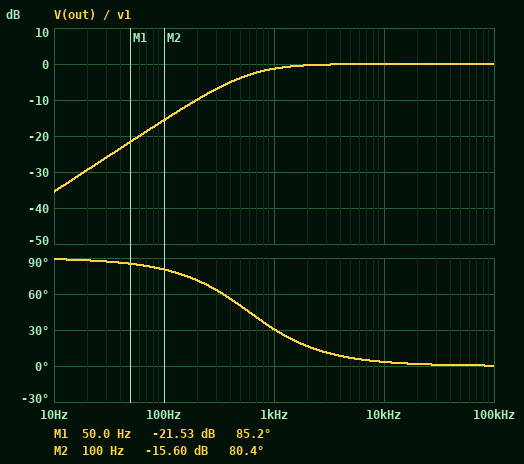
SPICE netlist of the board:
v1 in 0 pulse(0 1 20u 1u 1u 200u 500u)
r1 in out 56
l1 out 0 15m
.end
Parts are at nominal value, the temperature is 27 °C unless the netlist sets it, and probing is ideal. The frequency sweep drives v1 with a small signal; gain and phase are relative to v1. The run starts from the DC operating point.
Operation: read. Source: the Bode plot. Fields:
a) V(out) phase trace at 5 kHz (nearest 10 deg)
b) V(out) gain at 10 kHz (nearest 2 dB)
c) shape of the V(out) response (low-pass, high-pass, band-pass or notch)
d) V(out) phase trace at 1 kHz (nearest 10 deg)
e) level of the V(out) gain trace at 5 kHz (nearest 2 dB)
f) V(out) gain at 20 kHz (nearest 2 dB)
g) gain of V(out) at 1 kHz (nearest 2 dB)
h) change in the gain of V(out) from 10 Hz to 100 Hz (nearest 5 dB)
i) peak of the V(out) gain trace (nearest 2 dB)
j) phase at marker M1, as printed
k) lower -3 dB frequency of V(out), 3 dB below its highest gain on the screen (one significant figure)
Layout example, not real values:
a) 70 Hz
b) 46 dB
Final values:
a) 10 deg
b) 0 dB
c) high-pass
d) 30 deg
e) 0 dB
f) 0 dB
g) -2 dB
h) 20 dB
i) 0 dB
j) 85.2 deg
k) 600 Hz
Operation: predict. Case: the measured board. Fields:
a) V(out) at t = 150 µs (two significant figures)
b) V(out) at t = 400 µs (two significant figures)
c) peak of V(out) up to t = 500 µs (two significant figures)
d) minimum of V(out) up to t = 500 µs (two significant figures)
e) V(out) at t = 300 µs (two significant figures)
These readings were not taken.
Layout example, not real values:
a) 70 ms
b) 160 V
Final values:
a) 620 mV
b) -270 mV
c) 1.0 V
d) -530 mV
e) -390 mV
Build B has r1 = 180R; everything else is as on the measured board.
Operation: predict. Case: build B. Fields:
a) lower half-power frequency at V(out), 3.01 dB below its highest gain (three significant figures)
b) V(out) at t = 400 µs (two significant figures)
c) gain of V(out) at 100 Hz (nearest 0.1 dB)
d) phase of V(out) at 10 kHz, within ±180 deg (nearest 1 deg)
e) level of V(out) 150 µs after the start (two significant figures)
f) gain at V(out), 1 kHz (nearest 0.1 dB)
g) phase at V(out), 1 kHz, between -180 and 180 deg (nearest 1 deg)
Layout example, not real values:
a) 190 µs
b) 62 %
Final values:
a) 1.91 kHz
b) -110 mV
c) -25.6 dB
d) 11 deg
e) 210 mV
f) -6.7 dB
g) 62 deg
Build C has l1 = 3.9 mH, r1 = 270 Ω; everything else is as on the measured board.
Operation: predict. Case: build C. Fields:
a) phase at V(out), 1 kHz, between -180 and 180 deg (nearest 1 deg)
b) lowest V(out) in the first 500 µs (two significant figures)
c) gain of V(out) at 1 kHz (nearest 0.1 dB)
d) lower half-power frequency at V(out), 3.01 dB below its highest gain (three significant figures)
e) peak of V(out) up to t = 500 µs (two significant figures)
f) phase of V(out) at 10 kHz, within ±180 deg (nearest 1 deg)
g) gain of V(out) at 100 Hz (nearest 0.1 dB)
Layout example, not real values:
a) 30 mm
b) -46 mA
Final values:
a) 85 deg
b) -970 mV
c) -20.9 dB
d) 11.0 kHz
e) 970 mV
f) 48 deg
g) -40.8 dB
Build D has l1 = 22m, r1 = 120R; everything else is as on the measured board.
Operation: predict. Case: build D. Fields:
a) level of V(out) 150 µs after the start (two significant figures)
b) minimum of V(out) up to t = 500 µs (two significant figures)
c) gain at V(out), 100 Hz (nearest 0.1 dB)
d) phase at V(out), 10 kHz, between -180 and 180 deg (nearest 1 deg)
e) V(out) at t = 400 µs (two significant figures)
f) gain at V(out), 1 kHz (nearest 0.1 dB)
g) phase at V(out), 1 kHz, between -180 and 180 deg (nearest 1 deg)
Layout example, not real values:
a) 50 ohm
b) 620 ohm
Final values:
a) 490 mV
b) -660 mV
c) -18.8 dB
d) 5 deg
e) -250 mV
f) -2.4 dB
g) 41 deg
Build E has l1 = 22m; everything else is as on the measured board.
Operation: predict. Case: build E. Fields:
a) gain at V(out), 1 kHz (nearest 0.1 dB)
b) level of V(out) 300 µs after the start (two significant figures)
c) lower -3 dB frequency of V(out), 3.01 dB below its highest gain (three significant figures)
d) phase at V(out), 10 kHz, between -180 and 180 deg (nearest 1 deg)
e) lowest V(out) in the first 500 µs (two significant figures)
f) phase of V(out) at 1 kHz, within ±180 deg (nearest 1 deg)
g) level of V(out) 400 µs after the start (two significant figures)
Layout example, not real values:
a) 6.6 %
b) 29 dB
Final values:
a) -0.7 dB
b) -330 mV
c) 405 Hz
d) 2 deg
e) -400 mV
f) 22 deg
g) -250 mV
